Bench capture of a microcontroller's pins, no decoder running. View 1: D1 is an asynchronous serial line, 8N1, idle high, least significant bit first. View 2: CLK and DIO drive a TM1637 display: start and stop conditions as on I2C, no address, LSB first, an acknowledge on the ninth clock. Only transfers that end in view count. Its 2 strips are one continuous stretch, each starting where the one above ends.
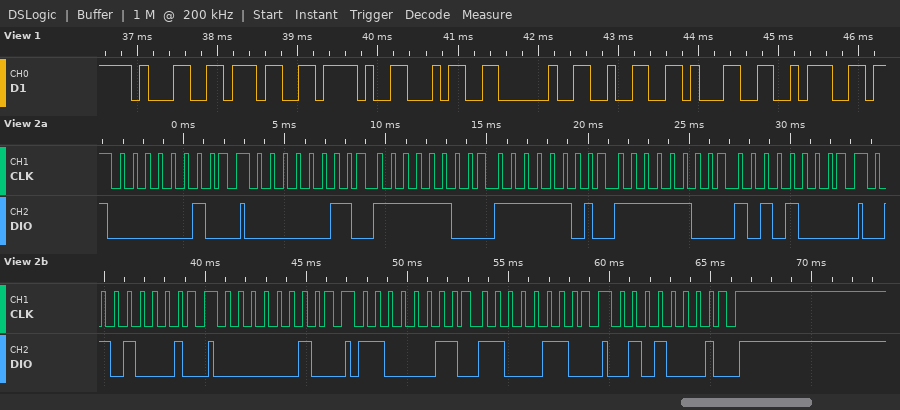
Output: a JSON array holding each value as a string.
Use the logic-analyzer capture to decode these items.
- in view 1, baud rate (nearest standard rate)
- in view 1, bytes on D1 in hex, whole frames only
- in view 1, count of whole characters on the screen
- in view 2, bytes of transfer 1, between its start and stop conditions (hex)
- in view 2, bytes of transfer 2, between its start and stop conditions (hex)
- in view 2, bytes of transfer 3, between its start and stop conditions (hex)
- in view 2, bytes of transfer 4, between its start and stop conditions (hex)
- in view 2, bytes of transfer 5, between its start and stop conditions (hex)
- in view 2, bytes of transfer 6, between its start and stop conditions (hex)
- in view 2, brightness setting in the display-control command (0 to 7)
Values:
["9600 baud", "31 37 2F 34 20 32 31 3A", "8", "40", "C0 3F BF 3F 15", "8A", "40", "C3 63", "8A", "2"]
